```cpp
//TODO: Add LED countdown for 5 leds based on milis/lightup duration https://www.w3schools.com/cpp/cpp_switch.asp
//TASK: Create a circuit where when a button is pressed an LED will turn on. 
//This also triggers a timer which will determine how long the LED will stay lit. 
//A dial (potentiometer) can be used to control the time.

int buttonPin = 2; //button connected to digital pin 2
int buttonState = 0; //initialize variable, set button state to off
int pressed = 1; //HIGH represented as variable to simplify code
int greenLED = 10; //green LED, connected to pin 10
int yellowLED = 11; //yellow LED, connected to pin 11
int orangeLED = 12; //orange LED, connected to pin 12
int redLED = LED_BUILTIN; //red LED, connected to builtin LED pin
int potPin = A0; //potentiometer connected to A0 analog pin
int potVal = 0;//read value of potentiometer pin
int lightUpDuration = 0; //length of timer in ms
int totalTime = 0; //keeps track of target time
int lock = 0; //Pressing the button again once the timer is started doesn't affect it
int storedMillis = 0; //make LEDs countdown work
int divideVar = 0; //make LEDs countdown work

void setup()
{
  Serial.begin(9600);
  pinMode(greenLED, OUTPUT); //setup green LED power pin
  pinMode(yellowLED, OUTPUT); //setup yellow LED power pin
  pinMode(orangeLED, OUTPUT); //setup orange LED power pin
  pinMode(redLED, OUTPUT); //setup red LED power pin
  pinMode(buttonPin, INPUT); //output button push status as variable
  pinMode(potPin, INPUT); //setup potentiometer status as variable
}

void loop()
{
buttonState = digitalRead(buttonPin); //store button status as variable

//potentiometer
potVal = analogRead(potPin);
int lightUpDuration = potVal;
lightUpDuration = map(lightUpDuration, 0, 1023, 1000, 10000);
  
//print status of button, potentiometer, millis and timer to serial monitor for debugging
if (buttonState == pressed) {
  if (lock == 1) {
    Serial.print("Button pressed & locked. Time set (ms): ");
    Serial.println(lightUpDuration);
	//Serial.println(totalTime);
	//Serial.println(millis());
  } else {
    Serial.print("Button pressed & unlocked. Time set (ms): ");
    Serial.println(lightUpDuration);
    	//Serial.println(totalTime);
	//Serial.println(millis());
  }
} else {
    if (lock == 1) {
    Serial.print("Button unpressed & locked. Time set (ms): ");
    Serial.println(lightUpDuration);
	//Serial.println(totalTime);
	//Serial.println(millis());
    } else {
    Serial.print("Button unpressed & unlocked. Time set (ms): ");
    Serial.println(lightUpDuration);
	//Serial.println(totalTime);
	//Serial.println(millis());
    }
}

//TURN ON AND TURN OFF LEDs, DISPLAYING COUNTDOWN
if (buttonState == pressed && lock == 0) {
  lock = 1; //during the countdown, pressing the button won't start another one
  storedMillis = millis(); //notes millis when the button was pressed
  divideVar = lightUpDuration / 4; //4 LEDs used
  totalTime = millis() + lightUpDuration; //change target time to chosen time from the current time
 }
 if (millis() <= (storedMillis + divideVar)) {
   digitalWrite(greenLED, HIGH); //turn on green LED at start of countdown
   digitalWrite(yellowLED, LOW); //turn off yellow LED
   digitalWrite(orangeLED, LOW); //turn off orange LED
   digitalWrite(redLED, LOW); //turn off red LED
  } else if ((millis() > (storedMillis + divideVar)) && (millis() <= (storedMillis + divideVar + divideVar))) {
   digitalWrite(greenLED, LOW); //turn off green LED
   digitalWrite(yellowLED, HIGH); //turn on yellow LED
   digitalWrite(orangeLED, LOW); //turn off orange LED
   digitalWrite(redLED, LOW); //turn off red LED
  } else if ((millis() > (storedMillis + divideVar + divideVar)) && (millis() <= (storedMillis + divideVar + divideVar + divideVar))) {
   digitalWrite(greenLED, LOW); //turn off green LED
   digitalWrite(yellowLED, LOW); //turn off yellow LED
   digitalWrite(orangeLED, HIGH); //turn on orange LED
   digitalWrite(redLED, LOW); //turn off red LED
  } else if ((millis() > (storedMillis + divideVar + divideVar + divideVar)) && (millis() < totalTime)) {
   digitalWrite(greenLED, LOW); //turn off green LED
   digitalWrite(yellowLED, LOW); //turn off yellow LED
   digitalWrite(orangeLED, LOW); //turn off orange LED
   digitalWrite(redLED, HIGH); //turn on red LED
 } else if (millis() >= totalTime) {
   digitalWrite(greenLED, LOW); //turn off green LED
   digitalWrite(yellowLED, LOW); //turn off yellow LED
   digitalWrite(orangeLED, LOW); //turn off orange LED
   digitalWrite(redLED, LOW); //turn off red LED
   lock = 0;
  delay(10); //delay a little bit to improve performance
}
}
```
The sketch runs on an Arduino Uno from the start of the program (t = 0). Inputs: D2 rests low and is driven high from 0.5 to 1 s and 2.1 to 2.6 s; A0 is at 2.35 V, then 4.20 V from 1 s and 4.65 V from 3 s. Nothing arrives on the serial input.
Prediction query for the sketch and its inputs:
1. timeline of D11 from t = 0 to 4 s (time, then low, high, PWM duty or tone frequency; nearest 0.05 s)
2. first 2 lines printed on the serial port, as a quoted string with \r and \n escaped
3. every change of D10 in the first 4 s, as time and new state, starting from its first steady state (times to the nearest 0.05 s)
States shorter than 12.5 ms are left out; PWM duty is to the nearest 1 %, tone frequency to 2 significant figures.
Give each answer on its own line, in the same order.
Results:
0 s low; 1.9 s high; 3.2 s low
"Button unpressed & unlocked. Time set (ms): 5231\r\nButton unpressed & unlocked. Time set (ms): 5231\r\n"
0 s high; 0.05 s low; 0.55 s high; 1.9 s low
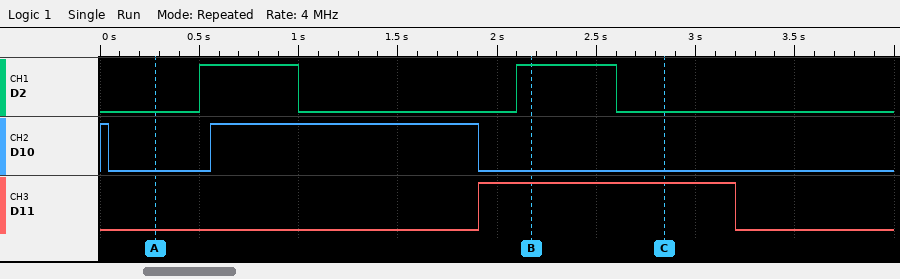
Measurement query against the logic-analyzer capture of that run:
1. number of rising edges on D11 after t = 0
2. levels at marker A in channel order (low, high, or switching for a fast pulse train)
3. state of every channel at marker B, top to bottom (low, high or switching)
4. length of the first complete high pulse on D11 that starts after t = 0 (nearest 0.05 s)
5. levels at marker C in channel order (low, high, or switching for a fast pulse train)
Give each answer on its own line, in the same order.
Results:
1
D2 low, D10 low, D11 low
D2 high, D10 low, D11 high
1.30 s
D2 low, D10 low, D11 high
